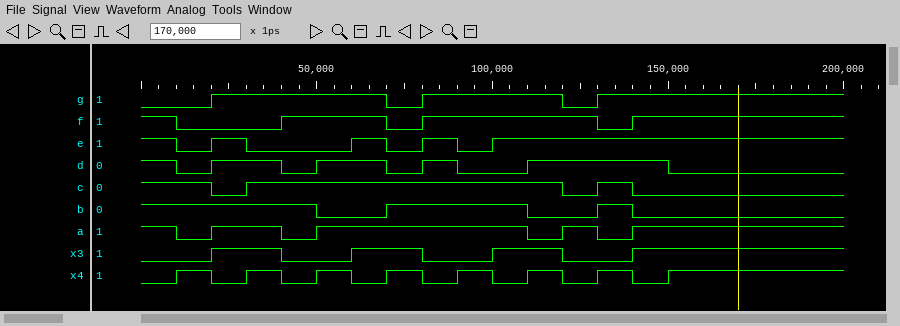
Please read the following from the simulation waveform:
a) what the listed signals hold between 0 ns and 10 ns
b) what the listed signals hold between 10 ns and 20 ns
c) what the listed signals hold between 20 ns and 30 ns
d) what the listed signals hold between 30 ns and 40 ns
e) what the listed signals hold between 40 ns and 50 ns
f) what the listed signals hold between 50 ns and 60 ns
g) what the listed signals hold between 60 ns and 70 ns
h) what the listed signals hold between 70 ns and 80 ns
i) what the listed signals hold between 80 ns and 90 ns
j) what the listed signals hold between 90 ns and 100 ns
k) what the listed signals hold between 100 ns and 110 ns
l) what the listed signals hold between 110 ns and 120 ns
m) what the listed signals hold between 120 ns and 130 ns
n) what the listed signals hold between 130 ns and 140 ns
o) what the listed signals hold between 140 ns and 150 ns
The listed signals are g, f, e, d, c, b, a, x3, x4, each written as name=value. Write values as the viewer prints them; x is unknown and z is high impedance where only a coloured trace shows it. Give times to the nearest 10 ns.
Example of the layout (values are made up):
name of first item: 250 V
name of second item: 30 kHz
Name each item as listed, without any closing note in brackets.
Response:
what the listed signals hold between 0 ns and 10 ns: g=0, f=1, e=1, d=1, c=1, b=1, a=1, x3=0, x4=0
what the listed signals hold between 10 ns and 20 ns: g=0, f=0, e=0, d=0, c=1, b=1, a=0, x3=0, x4=1
what the listed signals hold between 20 ns and 30 ns: g=1, f=0, e=1, d=1, c=0, b=1, a=1, x3=1, x4=0
what the listed signals hold between 30 ns and 40 ns: g=1, f=0, e=0, d=1, c=1, b=1, a=1, x3=1, x4=1
what the listed signals hold between 40 ns and 50 ns: g=1, f=1, e=0, d=0, c=1, b=1, a=0, x3=0, x4=0
what the listed signals hold between 50 ns and 60 ns: g=1, f=1, e=0, d=1, c=1, b=0, a=1, x3=0, x4=1
what the listed signals hold between 60 ns and 70 ns: g=1, f=1, e=1, d=1, c=1, b=0, a=1, x3=1, x4=0
what the listed signals hold between 70 ns and 80 ns: g=0, f=0, e=0, d=0, c=1, b=1, a=1, x3=1, x4=1
what the listed signals hold between 80 ns and 90 ns: g=1, f=1, e=1, d=1, c=1, b=1, a=1, x3=0, x4=0
what the listed signals hold between 90 ns and 100 ns: g=1, f=1, e=0, d=0, c=1, b=1, a=1, x3=0, x4=1
what the listed signals hold between 100 ns and 110 ns: g=1, f=1, e=1, d=0, c=1, b=1, a=1, x3=1, x4=0
what the listed signals hold between 110 ns and 120 ns: g=1, f=1, e=1, d=1, c=1, b=0, a=0, x3=1, x4=1
what the listed signals hold between 120 ns and 130 ns: g=0, f=1, e=1, d=1, c=0, b=0, a=1, x3=0, x4=0
what the listed signals hold between 130 ns and 140 ns: g=1, f=0, e=1, d=1, c=1, b=1, a=0, x3=0, x4=1
what the listed signals hold between 140 ns and 150 ns: g=1, f=1, e=1, d=1, c=0, b=0, a=1, x3=1, x4=0
